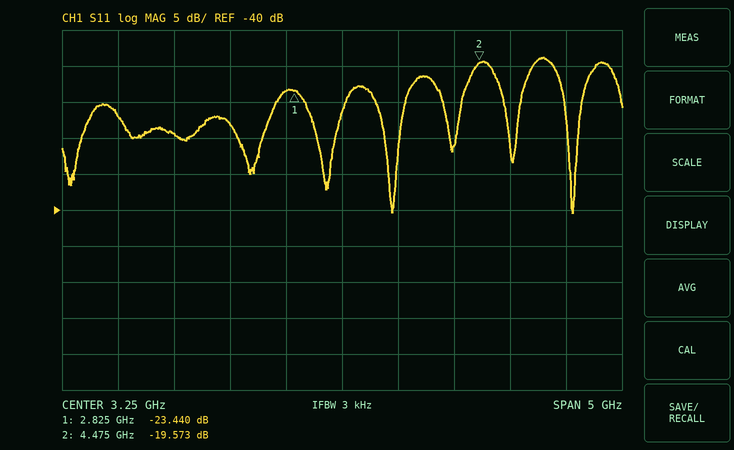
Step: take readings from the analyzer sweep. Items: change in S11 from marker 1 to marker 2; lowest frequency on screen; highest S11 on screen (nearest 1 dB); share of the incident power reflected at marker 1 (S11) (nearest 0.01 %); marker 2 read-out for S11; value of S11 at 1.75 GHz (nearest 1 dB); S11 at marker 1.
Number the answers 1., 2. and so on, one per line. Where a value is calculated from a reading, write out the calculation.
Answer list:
1. -19.573 − (-23.44) = 3.867 dB
2. 750 MHz
3. -19 dB
4. 10^(-23.44/10) ≈ 0.45 %
5. -19.573 dB
6. -29 dB
7. -23.440 dB
